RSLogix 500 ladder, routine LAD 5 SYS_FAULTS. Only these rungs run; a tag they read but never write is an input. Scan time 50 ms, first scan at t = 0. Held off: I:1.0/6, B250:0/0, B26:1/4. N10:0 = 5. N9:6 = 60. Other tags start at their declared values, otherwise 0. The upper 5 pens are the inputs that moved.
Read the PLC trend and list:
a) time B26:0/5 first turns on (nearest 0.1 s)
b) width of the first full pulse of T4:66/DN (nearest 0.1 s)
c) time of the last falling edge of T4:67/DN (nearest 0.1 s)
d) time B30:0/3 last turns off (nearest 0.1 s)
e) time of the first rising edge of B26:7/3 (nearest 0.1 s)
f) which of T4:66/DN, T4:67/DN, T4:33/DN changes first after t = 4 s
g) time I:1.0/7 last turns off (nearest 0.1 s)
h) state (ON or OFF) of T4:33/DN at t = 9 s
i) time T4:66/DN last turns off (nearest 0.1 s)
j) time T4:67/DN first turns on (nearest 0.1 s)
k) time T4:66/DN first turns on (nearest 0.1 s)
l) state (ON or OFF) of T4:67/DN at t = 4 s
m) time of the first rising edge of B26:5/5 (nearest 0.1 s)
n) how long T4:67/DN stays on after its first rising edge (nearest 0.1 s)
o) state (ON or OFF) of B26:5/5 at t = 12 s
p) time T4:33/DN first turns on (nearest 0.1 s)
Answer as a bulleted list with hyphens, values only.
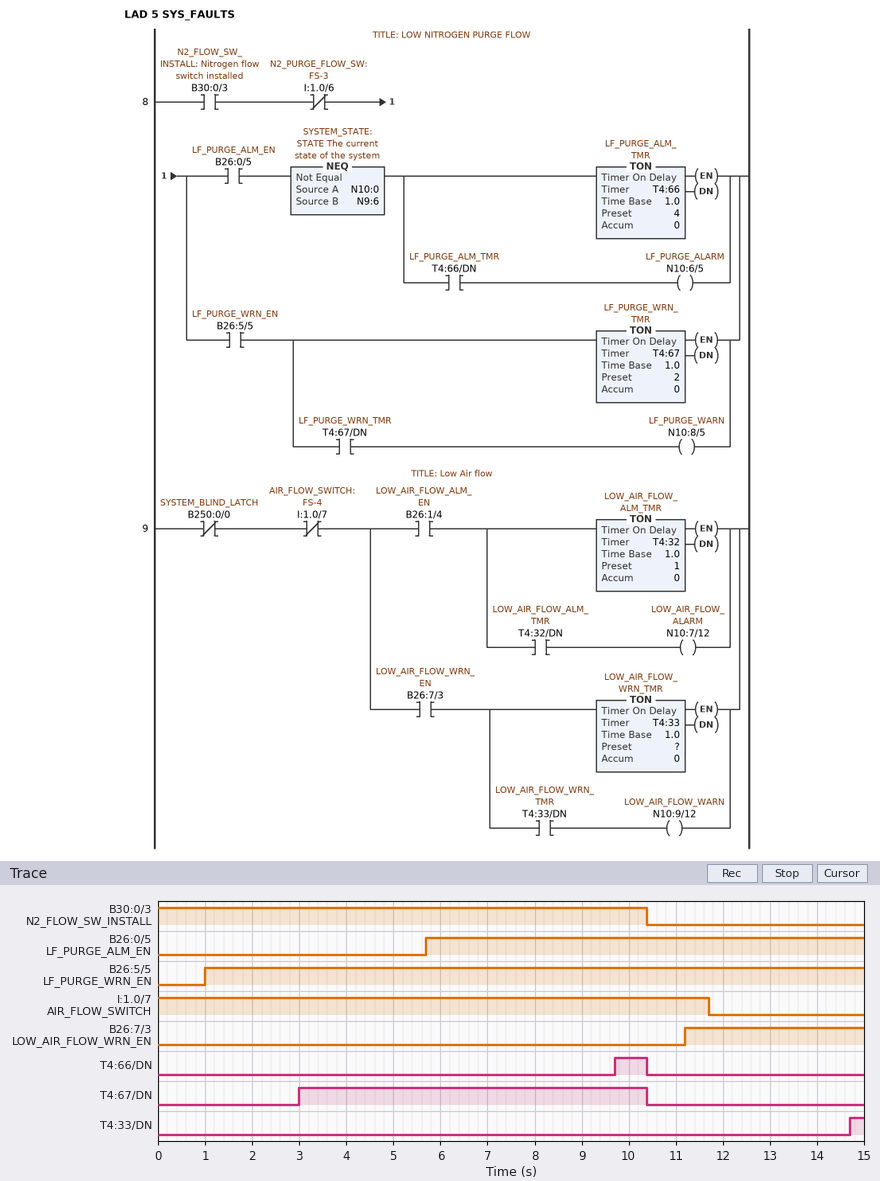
- 5.7 s
- 0.7 s
- 10.4 s
- 10.4 s
- 11.2 s
- T4:66/DN
- 11.7 s
- OFF
- 10.4 s
- 3.0 s
- 9.7 s
- ON
- 1.0 s
- 7.4 s
- ON
- 14.7 s
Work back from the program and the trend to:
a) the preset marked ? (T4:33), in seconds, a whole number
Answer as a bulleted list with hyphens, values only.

- 3 s
